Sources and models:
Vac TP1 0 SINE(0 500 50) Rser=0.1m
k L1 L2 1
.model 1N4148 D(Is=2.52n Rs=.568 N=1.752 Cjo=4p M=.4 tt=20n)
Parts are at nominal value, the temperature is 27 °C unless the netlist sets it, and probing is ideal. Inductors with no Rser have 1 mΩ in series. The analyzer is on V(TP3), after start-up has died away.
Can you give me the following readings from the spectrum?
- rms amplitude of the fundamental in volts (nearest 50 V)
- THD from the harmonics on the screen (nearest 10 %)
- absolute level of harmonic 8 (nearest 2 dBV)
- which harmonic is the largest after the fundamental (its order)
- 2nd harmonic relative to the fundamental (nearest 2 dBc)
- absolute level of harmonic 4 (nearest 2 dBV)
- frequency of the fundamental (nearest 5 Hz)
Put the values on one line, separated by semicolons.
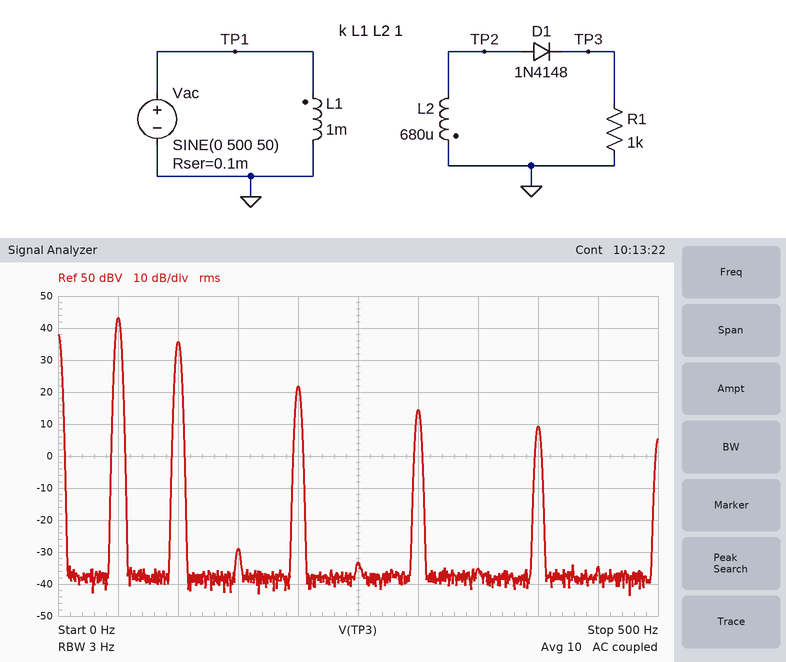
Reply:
150 V; 40 %; 10 dBV; 2; -8 dBc; 22 dBV; 50 Hz
